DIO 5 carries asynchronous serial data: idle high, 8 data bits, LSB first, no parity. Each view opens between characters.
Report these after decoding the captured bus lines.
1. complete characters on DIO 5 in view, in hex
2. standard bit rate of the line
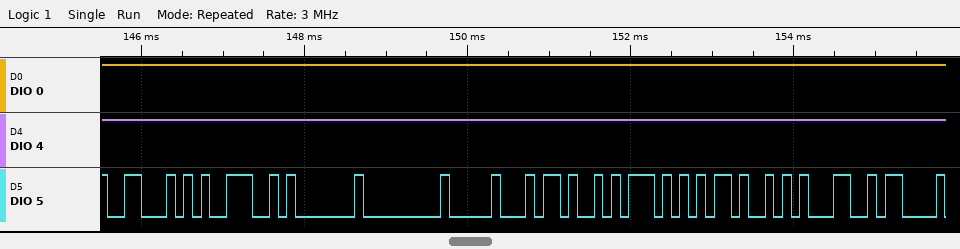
46, 39, 01, 00, 10, 4B, 57, 4B, 31
9600 baud
